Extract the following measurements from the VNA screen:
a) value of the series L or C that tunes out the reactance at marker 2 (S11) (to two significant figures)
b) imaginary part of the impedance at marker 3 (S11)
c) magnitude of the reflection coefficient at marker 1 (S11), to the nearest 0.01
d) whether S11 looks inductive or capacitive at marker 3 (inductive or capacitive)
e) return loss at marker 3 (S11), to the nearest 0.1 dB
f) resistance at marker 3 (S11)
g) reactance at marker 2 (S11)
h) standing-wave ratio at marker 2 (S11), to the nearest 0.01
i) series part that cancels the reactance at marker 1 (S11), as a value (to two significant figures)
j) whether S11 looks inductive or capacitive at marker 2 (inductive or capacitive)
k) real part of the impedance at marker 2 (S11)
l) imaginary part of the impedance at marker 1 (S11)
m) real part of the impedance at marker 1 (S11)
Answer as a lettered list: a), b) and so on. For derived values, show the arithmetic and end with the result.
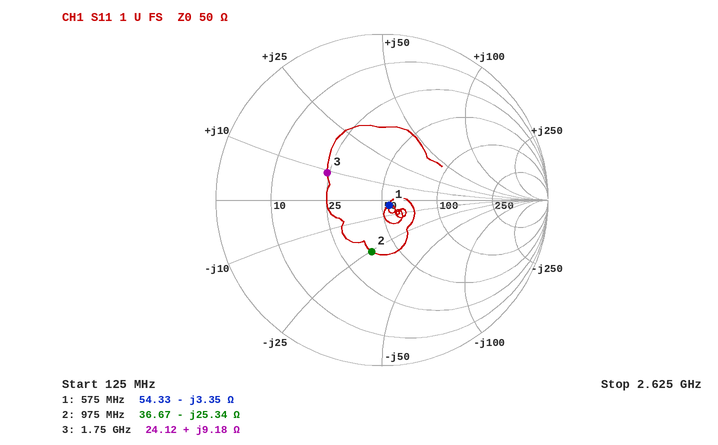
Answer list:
a) L = 25.34 Ω/(2π × 975 MHz) ≈ 4.1 nH
b) +9.18 Ω
c) 0.05
d) inductive
e) 8.7 dB
f) 24.12 Ω
g) -25.34 Ω
h) 1.93
i) L = 3.35 Ω/(2π × 575 MHz) ≈ 927 pH, so 930 pH to two significant figures
j) capacitive
k) 36.67 Ω
l) -3.35 Ω
m) 54.33 Ω
